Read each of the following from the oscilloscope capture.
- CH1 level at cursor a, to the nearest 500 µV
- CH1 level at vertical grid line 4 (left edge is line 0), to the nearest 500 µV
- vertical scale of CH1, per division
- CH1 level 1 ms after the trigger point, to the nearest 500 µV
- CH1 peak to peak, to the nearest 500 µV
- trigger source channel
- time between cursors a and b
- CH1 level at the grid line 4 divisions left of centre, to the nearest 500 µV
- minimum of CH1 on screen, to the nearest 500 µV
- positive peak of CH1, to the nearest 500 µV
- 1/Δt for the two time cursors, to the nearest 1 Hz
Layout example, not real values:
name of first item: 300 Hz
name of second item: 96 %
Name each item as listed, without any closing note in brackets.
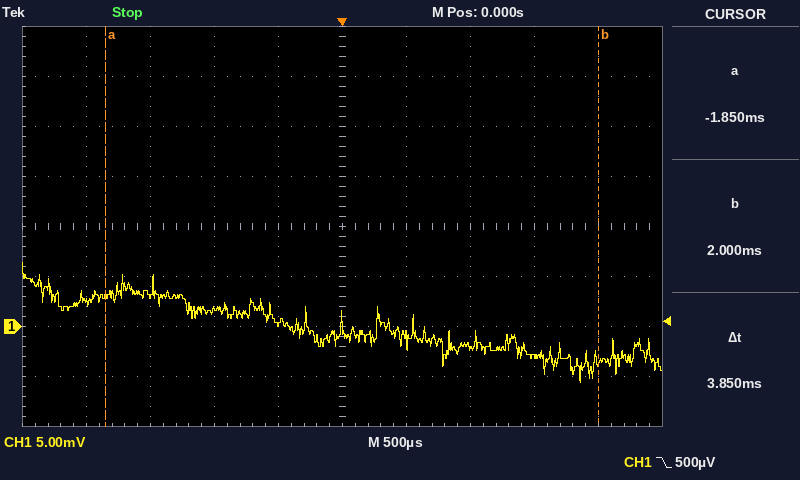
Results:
CH1 level at cursor a, to the nearest 500 µV: 3.0 mV
CH1 level at vertical grid line 4 (left edge is line 0), to the nearest 500 µV: 500 µV
vertical scale of CH1, per division: 5 mV
CH1 level 1 ms after the trigger point, to the nearest 500 µV: -2.0 mV
CH1 peak to peak, to the nearest 500 µV: 12.0 mV
trigger source channel: CH1
time between cursors a and b: 3.85 ms
CH1 level at the grid line 4 divisions left of centre, to the nearest 500 µV: 2.5 mV
minimum of CH1 on screen, to the nearest 500 µV: -5.5 mV
positive peak of CH1, to the nearest 500 µV: 6.5 mV
1/Δt for the two time cursors, to the nearest 1 Hz: 260 Hz
